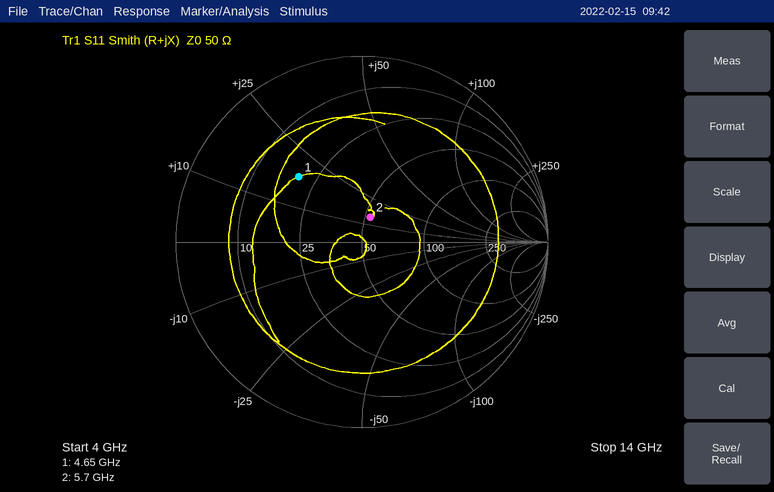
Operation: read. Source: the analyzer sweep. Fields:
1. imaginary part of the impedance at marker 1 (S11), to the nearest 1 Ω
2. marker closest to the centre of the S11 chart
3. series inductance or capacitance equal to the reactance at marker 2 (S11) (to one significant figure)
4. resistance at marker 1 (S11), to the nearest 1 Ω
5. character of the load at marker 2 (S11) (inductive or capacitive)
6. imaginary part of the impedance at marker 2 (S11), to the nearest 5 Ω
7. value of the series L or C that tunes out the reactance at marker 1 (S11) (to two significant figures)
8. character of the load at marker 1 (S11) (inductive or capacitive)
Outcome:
+18 Ω
marker 2
400 pH
20 Ω
inductive
+15 Ω
1.9 pF
inductive
